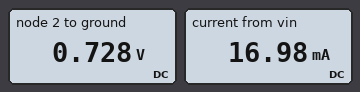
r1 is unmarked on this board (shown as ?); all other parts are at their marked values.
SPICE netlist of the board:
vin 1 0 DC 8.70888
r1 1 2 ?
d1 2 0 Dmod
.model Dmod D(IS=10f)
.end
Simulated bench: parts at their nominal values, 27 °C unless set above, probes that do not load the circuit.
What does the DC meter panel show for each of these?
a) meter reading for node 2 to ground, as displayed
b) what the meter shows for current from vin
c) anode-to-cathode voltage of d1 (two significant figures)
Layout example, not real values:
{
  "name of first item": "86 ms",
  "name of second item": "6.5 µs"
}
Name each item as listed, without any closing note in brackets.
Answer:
{
  "meter reading for node 2 to ground, as displayed": "0.728 V",
  "what the meter shows for current from vin": "16.98 mA",
  "anode-to-cathode voltage of d1": "730 mV"
}
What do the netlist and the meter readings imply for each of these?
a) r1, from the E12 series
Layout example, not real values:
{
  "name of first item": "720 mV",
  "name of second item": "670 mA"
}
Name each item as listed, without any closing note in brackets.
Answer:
{
  "r1, from the E12 series": "470 Ω"
}
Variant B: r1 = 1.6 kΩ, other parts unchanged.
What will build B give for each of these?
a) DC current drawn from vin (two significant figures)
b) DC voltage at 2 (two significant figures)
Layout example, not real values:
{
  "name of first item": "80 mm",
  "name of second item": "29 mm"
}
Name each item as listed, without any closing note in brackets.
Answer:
{
  "DC current drawn from vin": "5.0 mA",
  "DC voltage at 2": "700 mV"
}
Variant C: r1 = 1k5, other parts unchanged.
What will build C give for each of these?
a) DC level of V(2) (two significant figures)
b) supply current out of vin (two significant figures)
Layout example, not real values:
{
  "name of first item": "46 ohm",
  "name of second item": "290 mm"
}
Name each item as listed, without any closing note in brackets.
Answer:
{
  "DC level of V(2)": "700 mV",
  "supply current out of vin": "5.3 mA"
}
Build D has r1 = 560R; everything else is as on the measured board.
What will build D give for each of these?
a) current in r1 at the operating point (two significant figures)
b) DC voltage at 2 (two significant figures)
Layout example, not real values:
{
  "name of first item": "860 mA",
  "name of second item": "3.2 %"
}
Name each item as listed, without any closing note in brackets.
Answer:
{
  "current in r1 at the operating point": "14 mA",
  "DC voltage at 2": "720 mV"
}
